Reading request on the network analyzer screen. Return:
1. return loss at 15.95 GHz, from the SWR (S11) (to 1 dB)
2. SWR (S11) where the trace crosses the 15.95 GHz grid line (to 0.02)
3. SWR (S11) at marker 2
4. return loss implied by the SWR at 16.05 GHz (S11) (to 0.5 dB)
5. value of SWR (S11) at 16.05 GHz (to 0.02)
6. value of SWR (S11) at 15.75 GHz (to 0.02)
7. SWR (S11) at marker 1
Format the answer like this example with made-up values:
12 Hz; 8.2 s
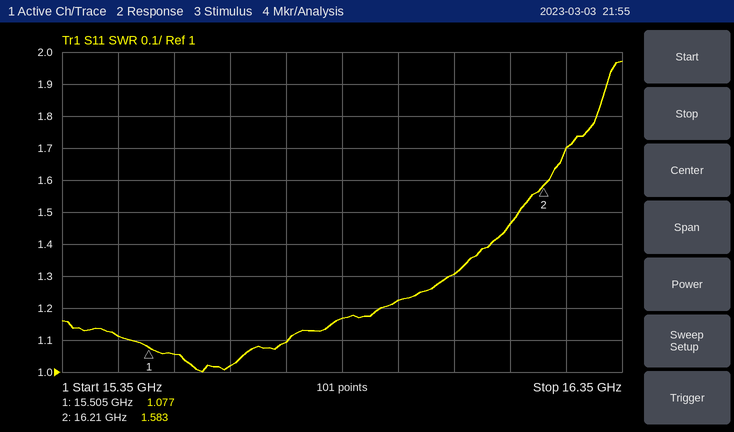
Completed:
20 dB; 1.22; 1.583; 17.5 dB; 1.30; 1.10; 1.077
